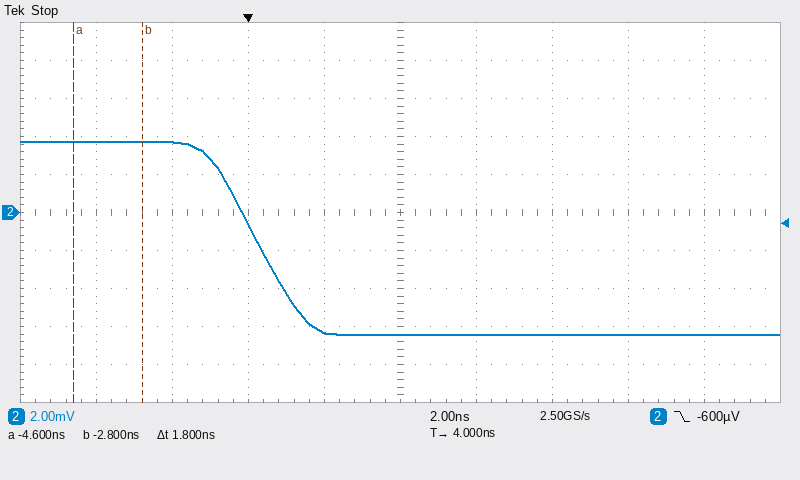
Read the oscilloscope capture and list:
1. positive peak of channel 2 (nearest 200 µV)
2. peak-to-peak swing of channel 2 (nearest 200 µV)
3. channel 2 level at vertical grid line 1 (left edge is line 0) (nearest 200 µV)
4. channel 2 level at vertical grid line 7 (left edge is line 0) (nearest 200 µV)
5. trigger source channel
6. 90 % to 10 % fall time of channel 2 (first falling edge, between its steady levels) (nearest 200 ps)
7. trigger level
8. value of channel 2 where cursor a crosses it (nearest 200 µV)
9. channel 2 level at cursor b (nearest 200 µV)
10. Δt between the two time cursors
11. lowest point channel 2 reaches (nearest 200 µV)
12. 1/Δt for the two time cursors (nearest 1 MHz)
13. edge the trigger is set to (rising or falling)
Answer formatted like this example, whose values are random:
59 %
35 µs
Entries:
3.8 mV
10.2 mV
3.8 mV
-6.4 mV
channel 2
2.4 ns
-600 µV
3.8 mV
3.8 mV
1.8 ns
-6.4 mV
556 MHz
falling
